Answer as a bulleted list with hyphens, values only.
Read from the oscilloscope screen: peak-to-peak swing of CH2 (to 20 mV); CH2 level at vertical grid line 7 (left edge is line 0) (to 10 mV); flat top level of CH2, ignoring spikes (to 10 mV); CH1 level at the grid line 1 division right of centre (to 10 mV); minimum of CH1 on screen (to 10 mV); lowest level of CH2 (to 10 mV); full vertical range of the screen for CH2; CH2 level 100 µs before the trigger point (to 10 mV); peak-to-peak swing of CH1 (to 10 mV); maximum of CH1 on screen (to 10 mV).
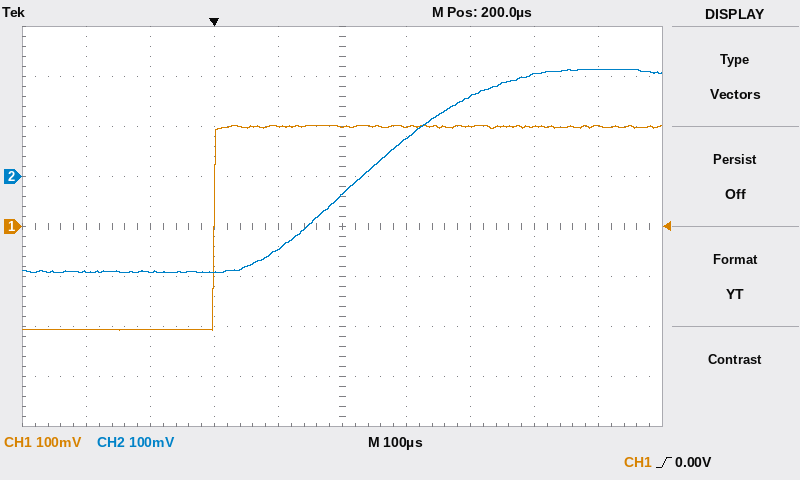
- 400 mV
- 160 mV
- 210 mV
- 200 mV
- -210 mV
- -190 mV
- 800 mV
- -190 mV
- 410 mV
- 200 mV
